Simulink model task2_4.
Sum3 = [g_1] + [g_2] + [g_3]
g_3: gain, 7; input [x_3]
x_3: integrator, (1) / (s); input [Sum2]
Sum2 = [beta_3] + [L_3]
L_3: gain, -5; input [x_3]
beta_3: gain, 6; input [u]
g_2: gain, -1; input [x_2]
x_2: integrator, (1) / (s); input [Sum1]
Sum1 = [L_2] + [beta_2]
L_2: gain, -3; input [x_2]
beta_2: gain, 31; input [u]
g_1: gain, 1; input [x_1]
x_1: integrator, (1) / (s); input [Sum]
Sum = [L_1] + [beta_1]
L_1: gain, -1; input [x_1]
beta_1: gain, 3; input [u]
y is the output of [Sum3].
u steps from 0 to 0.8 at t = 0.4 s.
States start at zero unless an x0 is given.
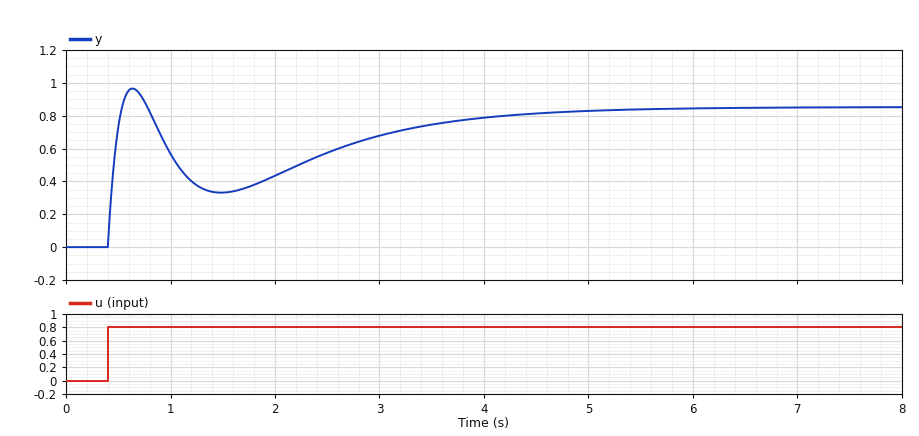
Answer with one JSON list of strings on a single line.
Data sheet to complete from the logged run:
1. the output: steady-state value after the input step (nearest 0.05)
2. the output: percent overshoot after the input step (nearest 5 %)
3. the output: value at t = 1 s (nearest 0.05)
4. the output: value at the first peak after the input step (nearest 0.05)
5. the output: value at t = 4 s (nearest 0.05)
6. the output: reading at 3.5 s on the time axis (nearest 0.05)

["0.85", "15 %", "0.55", "0.95", "0.80", "0.75"]
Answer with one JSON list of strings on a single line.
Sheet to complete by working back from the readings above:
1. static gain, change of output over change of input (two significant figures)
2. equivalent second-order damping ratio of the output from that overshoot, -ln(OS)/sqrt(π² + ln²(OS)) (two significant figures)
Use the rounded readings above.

["1.1", "0.52"]
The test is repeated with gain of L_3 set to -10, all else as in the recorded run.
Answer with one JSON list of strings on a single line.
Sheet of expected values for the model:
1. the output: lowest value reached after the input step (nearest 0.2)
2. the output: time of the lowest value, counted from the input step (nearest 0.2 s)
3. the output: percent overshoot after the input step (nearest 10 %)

["-3.0", "1.2 s", "20 %"]
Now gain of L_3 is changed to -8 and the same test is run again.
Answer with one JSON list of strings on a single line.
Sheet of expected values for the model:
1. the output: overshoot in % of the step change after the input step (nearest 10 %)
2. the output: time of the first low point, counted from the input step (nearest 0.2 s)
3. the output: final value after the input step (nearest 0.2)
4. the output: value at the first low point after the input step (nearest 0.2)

["30 %", "1.2 s", "-1.6", "-2.2"]
